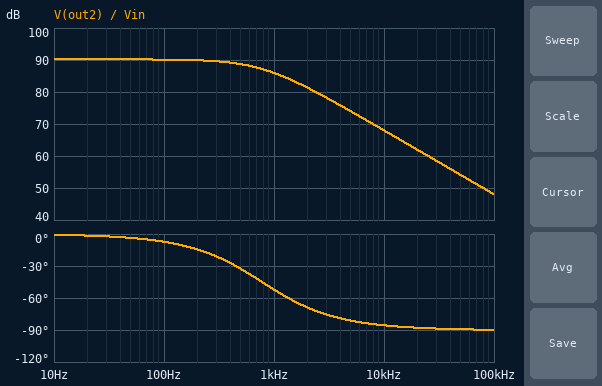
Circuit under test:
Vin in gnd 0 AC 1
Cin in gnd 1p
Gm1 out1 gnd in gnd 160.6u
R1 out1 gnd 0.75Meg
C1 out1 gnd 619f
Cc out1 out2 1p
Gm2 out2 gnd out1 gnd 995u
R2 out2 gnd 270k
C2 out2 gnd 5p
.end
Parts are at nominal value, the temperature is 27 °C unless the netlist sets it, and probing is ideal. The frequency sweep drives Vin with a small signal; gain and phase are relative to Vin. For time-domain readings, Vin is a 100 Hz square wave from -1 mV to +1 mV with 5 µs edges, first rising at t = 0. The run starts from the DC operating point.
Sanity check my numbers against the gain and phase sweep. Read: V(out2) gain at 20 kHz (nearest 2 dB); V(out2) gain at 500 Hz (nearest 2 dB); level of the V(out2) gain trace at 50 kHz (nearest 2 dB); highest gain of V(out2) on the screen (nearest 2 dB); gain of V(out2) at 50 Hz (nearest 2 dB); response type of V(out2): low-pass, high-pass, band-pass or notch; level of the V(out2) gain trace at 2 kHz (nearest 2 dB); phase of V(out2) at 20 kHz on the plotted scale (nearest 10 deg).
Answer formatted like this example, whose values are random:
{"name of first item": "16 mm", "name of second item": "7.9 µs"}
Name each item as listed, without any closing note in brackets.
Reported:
{"V(out2) gain at 20 kHz": "62 dB", "V(out2) gain at 500 Hz": "88 dB", "level of the V(out2) gain trace at 50 kHz": "54 dB", "highest gain of V(out2) on the screen": "90 dB", "gain of V(out2) at 50 Hz": "90 dB", "response type of V(out2): low-pass, high-pass, band-pass or notch": "low-pass", "level of the V(out2) gain trace at 2 kHz": "82 dB", "phase of V(out2) at 20 kHz on the plotted scale": "-90 deg"}
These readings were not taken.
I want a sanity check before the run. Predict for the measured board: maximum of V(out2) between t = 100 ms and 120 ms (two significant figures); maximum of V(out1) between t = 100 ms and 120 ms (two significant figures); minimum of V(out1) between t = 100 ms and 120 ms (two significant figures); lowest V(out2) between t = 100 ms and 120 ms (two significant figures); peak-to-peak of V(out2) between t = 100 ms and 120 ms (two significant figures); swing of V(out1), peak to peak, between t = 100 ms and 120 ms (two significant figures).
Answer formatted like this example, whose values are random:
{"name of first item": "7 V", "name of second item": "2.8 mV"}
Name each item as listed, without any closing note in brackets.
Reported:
{"maximum of V(out2) between t = 100 ms and 120 ms": "32 V", "maximum of V(out1) between t = 100 ms and 120 ms": "120 mV", "minimum of V(out1) between t = 100 ms and 120 ms": "-120 mV", "lowest V(out2) between t = 100 ms and 120 ms": "-32 V", "peak-to-peak of V(out2) between t = 100 ms and 120 ms": "65 V", "swing of V(out1), peak to peak, between t = 100 ms and 120 ms": "240 mV"}
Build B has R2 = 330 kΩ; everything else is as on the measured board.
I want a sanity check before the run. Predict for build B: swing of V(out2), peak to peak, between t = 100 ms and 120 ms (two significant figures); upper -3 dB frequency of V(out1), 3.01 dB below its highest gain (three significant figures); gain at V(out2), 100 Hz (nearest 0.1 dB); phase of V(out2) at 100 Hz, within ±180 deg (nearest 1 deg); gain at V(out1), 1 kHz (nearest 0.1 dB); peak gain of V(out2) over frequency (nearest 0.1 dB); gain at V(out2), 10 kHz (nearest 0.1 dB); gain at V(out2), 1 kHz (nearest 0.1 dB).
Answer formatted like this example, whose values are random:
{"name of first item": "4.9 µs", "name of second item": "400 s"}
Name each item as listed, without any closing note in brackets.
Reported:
{"swing of V(out2), peak to peak, between t = 100 ms and 120 ms": "79 V", "upper -3 dB frequency of V(out1), 3.01 dB below its highest gain": "638 Hz", "gain at V(out2), 100 Hz": "91.8 dB", "phase of V(out2) at 100 Hz, within ±180 deg": "-9 deg", "gain at V(out1), 1 kHz": "36.2 dB", "peak gain of V(out2) over frequency": "91.9 dB", "gain at V(out2), 10 kHz": "68.0 dB", "gain at V(out2), 1 kHz": "86.6 dB"}
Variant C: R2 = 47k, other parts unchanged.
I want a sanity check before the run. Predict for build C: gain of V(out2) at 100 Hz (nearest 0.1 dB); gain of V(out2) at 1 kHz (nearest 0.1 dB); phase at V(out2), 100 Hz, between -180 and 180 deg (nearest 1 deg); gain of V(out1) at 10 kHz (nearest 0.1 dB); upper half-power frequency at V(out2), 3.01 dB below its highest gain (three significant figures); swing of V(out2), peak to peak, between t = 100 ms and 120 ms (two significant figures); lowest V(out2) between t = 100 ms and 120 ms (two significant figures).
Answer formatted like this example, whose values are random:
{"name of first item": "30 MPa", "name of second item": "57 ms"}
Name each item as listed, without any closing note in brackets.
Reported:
{"gain of V(out2) at 100 Hz": "75.0 dB", "gain of V(out2) at 1 kHz": "74.8 dB", "phase at V(out2), 100 Hz, between -180 and 180 deg": "-1 deg", "gain of V(out1) at 10 kHz": "33.6 dB", "upper half-power frequency at V(out2), 3.01 dB below its highest gain": "4.35 kHz", "swing of V(out2), peak to peak, between t = 100 ms and 120 ms": "11 V", "lowest V(out2) between t = 100 ms and 120 ms": "-5.6 V"}
